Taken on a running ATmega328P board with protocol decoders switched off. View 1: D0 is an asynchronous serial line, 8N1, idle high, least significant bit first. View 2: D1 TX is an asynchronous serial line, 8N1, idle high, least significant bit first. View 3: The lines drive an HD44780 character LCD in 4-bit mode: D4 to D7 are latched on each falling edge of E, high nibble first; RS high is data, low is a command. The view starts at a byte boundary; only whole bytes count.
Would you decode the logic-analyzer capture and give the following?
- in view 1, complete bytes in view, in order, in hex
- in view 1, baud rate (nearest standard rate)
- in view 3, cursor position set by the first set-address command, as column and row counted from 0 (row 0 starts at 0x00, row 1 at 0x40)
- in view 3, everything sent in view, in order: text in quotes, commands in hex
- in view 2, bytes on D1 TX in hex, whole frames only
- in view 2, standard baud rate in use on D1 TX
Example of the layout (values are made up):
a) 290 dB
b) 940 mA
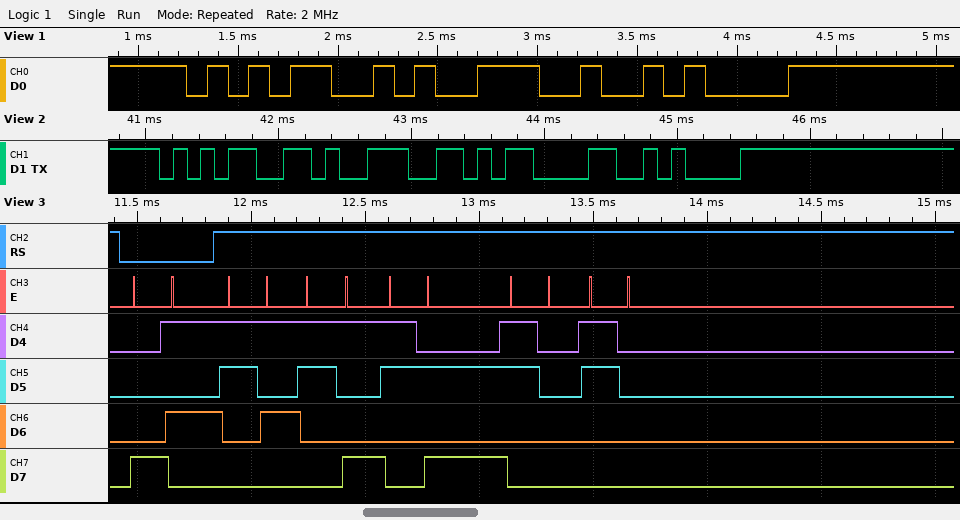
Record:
a) 35 39 0A
b) 9600 baud
c) column 5, row 0
d) 0x85 "59:00"
e) 35 39 0D 0A
f) 9600 baud
